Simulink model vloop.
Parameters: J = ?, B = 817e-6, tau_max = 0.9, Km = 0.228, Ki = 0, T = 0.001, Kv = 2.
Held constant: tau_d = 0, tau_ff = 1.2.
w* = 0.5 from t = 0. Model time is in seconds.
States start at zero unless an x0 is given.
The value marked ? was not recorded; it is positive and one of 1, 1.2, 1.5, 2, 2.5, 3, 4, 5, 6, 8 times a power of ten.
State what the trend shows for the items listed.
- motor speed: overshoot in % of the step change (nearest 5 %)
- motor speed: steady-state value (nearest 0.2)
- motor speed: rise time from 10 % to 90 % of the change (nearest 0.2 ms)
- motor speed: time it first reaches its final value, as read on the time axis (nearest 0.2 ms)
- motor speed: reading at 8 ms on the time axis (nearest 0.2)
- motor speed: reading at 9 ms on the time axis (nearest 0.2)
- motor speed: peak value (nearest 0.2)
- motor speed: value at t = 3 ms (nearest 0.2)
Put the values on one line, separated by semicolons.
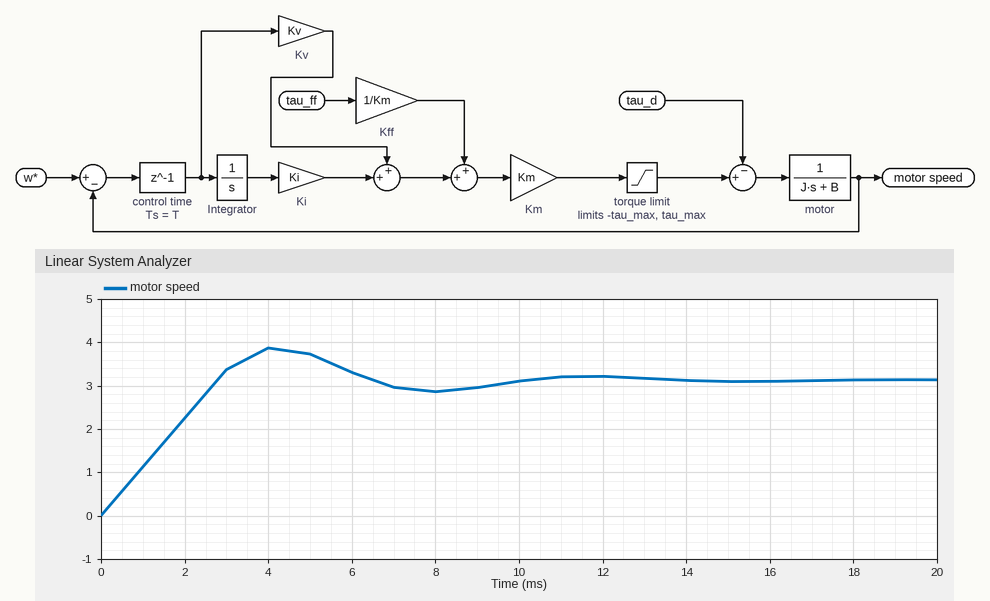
25 %; 3.2; 2.2 ms; 2.8 ms; 2.8; 3.0; 3.8; 3.4
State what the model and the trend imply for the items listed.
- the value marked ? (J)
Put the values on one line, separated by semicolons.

0.0008
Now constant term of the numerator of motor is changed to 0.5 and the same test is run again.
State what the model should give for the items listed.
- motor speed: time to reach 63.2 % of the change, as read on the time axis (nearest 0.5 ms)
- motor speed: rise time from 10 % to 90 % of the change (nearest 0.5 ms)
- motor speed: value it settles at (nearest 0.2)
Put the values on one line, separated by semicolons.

3.5 ms; 5.0 ms; 3.2
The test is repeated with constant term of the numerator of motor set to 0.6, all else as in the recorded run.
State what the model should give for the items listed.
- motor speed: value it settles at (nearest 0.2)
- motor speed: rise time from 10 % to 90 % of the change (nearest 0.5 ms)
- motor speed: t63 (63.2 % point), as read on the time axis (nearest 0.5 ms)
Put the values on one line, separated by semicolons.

3.2; 4.0 ms; 3.0 ms
